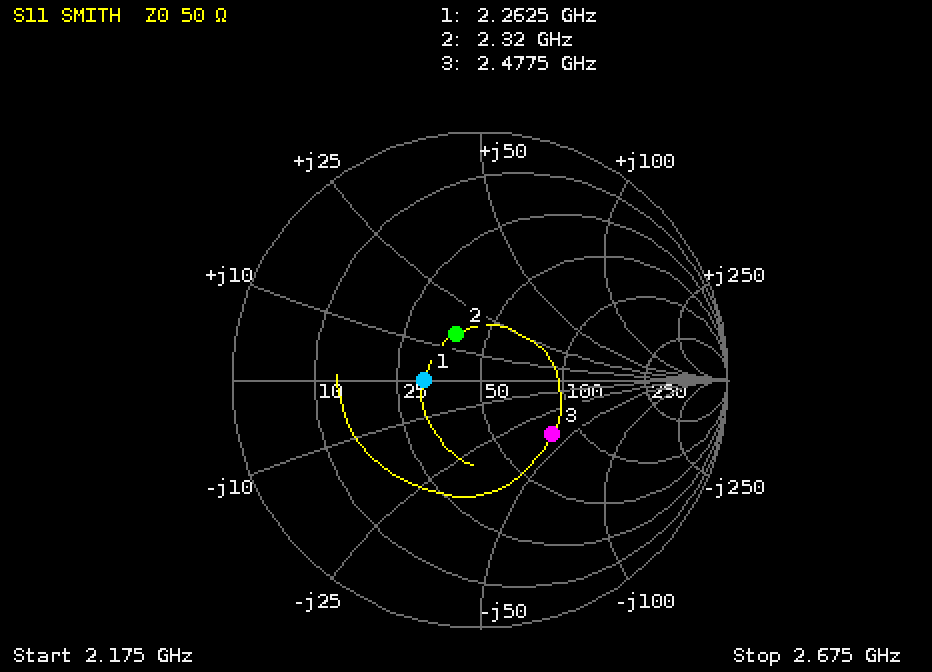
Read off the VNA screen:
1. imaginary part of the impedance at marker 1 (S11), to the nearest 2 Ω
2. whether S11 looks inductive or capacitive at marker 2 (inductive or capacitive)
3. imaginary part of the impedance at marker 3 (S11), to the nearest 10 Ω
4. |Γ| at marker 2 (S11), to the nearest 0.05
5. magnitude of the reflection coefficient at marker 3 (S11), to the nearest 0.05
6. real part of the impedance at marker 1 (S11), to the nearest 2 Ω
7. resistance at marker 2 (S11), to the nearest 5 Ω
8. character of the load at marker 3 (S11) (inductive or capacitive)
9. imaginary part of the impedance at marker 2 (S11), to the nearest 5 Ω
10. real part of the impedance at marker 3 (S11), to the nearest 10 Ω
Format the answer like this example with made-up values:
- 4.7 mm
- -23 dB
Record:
- 0 Ω
- inductive
- -40 Ω
- 0.20
- 0.35
- 32 Ω
- 40 Ω
- capacitive
- +15 Ω
- 80 Ω
